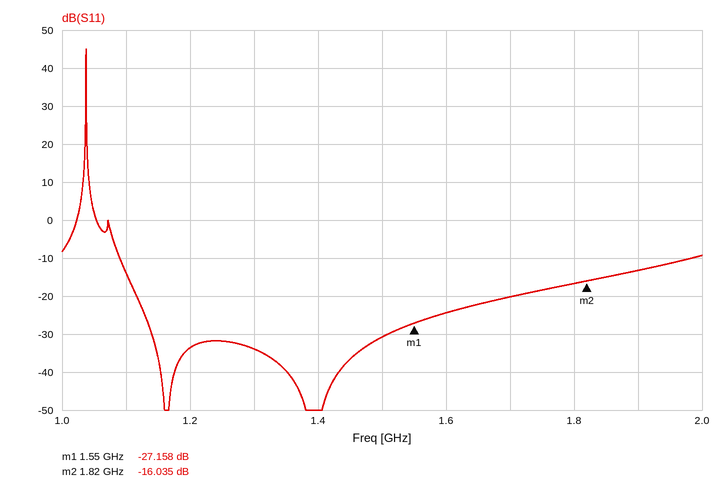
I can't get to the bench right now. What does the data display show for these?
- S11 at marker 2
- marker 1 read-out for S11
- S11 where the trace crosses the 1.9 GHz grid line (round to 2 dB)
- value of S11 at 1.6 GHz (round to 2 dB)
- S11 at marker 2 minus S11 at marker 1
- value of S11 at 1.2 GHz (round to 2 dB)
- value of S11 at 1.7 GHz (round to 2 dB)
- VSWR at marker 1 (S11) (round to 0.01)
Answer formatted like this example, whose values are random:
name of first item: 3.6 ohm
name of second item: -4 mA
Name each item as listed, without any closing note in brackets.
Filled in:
S11 at marker 2: -16.035 dB
marker 1 read-out for S11: -27.158 dB
S11 where the trace crosses the 1.9 GHz grid line: -14 dB
value of S11 at 1.6 GHz: -24 dB
S11 at marker 2 minus S11 at marker 1: 11.123 dB
value of S11 at 1.2 GHz: -34 dB
value of S11 at 1.7 GHz: -20 dB
VSWR at marker 1 (S11): 1.09
